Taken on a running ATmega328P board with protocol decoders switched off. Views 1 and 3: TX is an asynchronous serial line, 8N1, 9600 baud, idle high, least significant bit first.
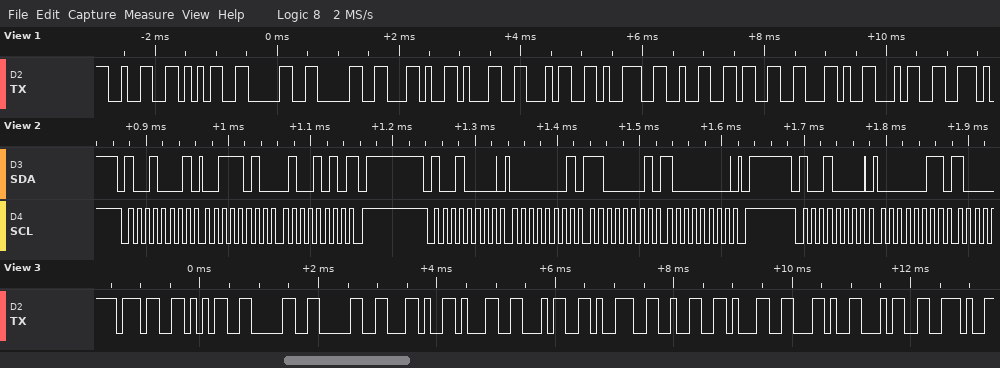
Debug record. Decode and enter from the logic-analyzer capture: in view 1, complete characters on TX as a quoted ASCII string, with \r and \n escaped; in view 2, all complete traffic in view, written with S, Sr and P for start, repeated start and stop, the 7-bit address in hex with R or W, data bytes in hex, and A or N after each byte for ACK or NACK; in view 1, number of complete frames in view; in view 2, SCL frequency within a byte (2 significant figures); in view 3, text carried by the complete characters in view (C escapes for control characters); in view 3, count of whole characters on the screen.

"2500,14923,4"
S 48R A 3A A 4A N P S 48W A 01 A C1 A 80 A P S 48W A 03 A
12
100 kHz
"7500,14921,4."
13
